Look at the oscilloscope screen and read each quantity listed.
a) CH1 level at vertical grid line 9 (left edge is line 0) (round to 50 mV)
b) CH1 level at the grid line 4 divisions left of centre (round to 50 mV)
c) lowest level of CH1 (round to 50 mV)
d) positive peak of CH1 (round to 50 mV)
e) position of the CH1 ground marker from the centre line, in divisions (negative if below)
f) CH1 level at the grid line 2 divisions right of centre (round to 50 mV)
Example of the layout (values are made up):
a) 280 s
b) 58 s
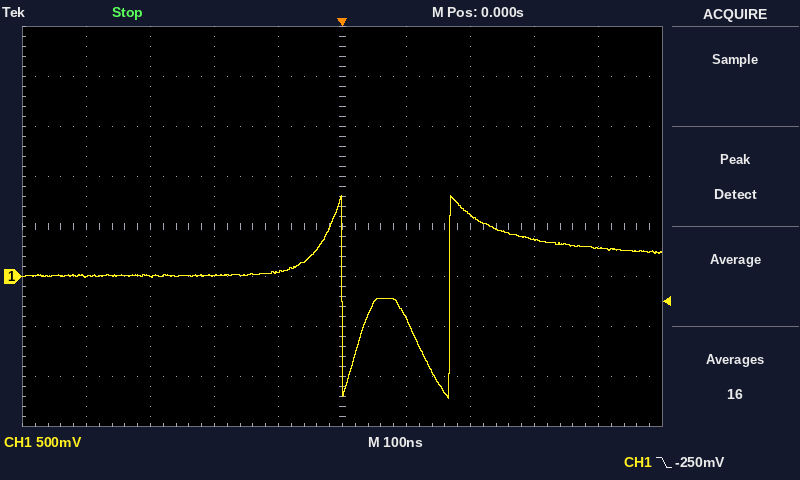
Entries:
a) 300 mV
b) 0 mV
c) -1.20 V
d) 800 mV
e) -1.0 div
f) 600 mV
